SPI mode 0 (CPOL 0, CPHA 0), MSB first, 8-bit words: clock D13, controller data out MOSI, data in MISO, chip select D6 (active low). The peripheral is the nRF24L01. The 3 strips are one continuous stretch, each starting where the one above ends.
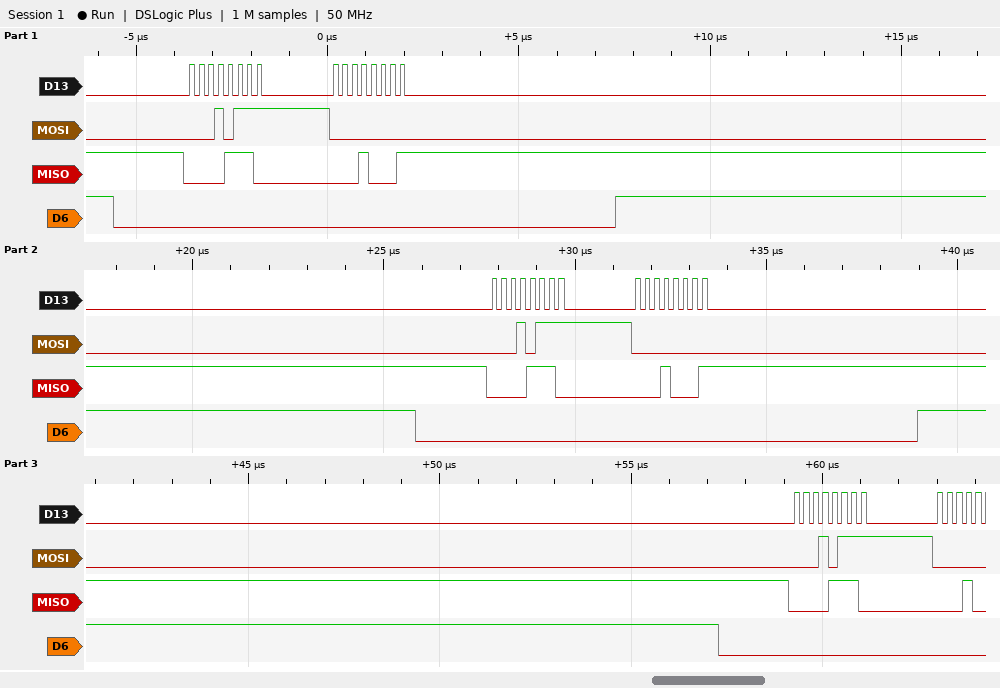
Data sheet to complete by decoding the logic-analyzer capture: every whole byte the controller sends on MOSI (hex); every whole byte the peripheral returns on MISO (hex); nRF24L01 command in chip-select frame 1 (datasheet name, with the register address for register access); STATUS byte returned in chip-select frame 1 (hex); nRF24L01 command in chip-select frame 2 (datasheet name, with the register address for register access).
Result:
0x17 0x00 0x17 0x00 0x17
0x0E 0x11 0x0E 0x11 0x0E
R_REGISTER 0x17
0x0E
R_REGISTER 0x17
